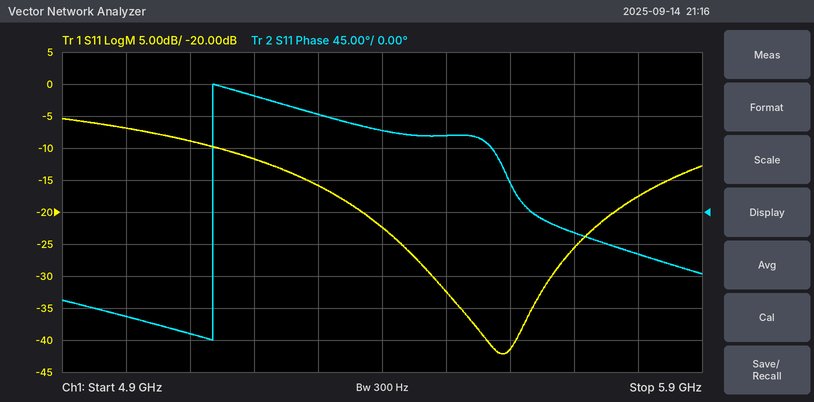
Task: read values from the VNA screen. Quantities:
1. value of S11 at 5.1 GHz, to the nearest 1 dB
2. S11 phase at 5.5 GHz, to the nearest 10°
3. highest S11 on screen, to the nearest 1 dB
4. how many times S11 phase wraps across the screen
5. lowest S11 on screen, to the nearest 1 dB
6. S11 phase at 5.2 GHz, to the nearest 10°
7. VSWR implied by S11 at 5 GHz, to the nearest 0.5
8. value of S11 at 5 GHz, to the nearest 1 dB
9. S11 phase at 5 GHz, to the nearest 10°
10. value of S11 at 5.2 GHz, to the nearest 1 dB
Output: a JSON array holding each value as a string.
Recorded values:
["-9 dB", "110°", "-5 dB", "1", "-42 dB", "160°", "2.5", "-7 dB", "-150°", "-12 dB"]
